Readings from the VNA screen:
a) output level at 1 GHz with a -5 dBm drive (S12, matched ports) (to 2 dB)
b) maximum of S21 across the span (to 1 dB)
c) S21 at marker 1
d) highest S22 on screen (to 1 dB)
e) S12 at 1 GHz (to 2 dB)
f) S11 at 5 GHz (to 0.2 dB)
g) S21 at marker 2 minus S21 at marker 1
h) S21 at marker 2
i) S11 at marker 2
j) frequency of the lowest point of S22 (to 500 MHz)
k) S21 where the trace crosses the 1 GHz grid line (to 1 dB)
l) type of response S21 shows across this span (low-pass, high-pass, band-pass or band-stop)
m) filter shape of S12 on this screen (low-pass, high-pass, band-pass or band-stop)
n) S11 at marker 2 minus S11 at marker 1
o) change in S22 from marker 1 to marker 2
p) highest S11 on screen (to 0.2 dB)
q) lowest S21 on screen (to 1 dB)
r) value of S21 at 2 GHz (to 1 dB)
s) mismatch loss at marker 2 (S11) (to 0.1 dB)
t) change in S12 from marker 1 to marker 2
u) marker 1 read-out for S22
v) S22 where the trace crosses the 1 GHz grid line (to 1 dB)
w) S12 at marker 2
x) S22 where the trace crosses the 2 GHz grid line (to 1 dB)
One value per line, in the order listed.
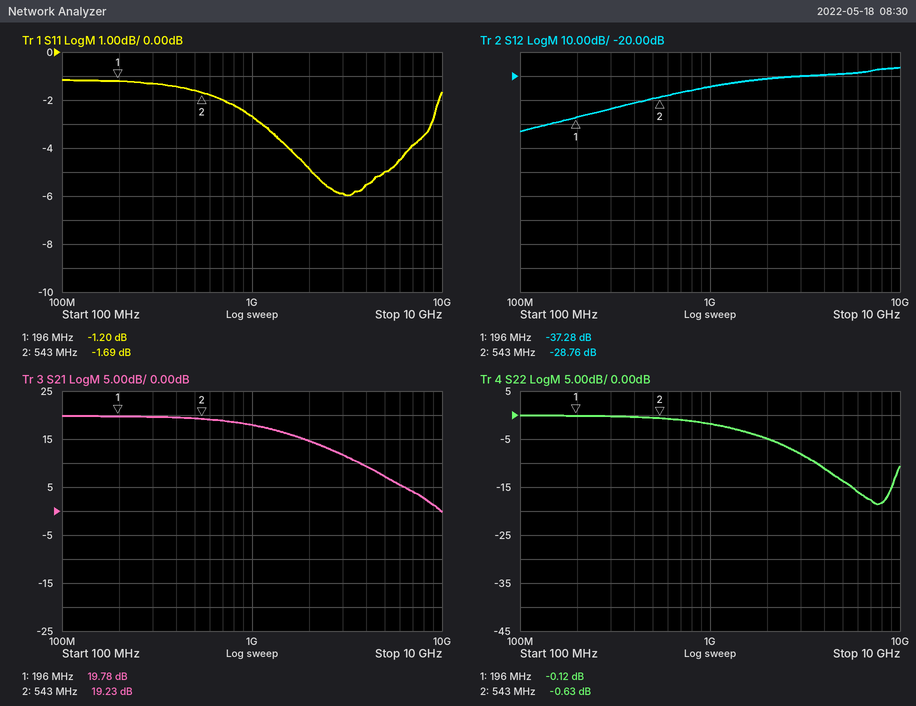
-30 dBm
20 dB
19.78 dB
0 dB
-24 dB
-5.0 dB
-0.55 dB
19.23 dB
-1.69 dB
7.5 GHz
18 dB
low-pass
high-pass
-0.49 dB
-0.51 dB
-1.2 dB
0 dB
15 dB
4.9 dB
8.52 dB
-0.12 dB
-2 dB
-28.76 dB
-5 dB
